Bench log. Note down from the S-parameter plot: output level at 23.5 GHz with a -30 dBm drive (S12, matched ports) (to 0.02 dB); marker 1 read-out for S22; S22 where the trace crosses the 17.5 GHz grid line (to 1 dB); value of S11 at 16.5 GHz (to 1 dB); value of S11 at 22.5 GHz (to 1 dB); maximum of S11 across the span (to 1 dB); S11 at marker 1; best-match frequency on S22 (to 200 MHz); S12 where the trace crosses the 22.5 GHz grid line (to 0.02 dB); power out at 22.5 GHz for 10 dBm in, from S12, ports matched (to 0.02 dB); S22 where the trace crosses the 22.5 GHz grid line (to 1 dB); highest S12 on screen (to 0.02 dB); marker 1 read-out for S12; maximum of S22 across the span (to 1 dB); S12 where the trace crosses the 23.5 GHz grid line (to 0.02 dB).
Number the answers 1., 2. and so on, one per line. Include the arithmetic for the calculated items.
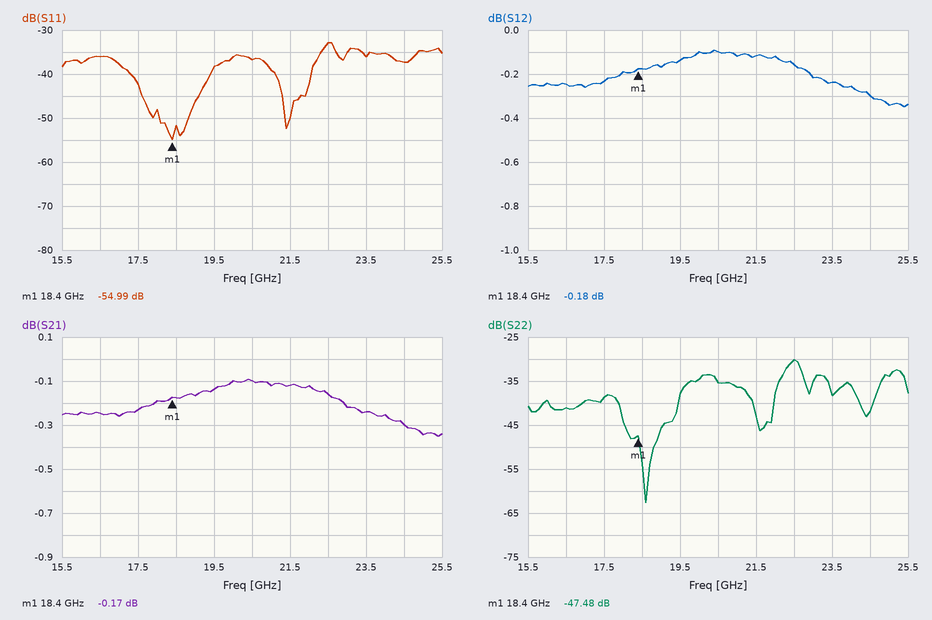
1. -30 dBm + (-0.24 dB) = -30.24 dBm
2. -47.48 dB
3. -39 dB
4. -36 dB
5. -33 dB
6. -33 dB
7. -54.99 dB
8. 18.6 GHz
9. -0.16 dB
10. 10 dBm + (-0.16 dB) = 9.84 dBm
11. -30 dB
12. -0.10 dB
13. -0.18 dB
14. -30 dB
15. -0.24 dB
